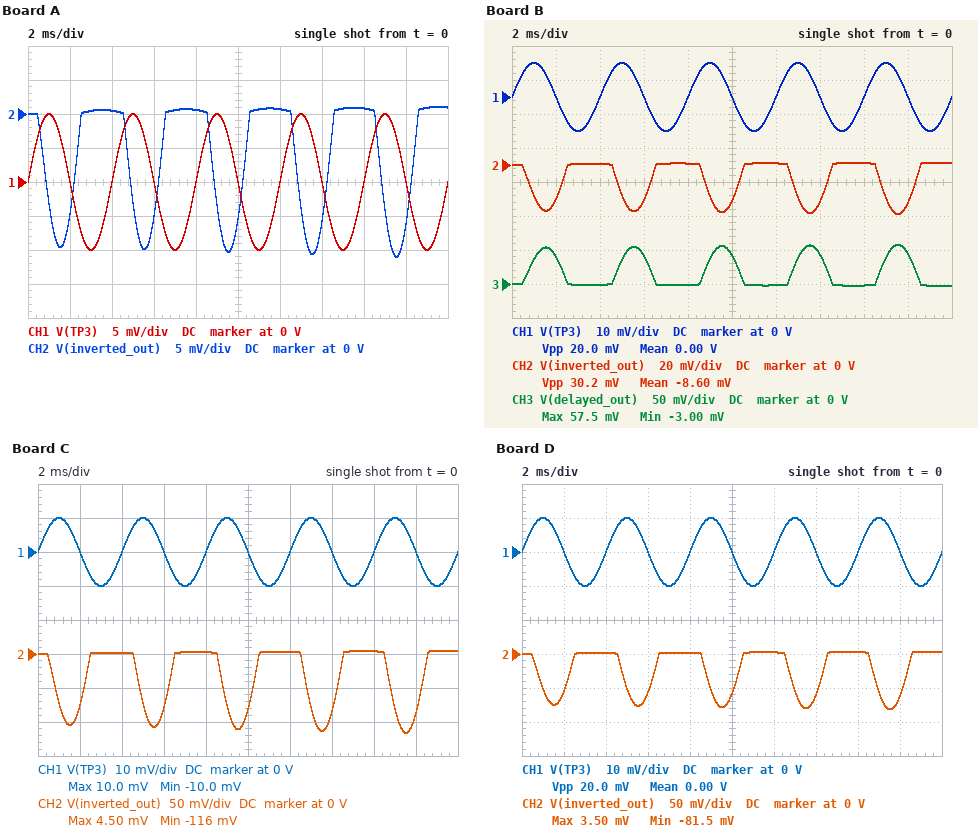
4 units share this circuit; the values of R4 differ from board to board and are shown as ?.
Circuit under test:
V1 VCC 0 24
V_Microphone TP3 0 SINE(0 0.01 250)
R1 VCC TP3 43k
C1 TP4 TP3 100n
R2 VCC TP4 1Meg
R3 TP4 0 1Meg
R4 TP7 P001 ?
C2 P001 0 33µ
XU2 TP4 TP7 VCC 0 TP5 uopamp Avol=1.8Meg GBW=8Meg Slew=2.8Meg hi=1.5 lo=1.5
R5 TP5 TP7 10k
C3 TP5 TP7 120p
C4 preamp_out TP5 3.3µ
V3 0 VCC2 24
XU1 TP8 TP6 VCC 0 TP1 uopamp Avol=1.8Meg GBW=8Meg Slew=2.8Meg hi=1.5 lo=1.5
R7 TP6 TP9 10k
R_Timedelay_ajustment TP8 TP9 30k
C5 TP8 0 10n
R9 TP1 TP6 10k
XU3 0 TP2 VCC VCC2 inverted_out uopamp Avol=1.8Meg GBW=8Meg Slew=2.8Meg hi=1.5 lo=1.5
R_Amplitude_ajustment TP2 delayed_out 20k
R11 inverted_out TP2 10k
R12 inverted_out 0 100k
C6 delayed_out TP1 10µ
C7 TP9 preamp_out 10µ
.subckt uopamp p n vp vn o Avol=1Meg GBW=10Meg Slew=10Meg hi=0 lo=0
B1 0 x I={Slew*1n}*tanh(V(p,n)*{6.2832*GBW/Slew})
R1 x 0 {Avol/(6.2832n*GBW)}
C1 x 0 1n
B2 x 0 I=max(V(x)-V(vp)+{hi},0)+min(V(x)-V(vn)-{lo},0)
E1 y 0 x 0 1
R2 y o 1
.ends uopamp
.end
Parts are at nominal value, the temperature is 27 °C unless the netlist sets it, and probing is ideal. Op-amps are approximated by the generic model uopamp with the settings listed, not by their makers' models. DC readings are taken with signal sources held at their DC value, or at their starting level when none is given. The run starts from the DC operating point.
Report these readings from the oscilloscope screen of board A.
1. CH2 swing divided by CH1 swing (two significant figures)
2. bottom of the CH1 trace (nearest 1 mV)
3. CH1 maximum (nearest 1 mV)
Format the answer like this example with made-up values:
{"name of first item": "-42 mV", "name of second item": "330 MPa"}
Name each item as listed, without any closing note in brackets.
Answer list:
{"CH2 swing divided by CH1 swing": "1.1", "bottom of the CH1 trace": "-10 mV", "CH1 maximum": "10 mV"}
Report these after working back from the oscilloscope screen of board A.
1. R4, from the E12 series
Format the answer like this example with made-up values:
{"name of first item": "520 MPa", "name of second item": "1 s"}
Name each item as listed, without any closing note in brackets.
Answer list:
{"R4, from the E12 series": "3.3 kΩ"}
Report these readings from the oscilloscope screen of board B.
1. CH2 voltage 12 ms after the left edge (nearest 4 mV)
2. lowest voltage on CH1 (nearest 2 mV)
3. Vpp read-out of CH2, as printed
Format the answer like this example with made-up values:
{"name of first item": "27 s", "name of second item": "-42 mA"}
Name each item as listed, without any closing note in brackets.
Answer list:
{"CH2 voltage 12 ms after the left edge": "0 V", "lowest voltage on CH1": "-10 mV", "Vpp read-out of CH2, as printed": "30.2 mV"}
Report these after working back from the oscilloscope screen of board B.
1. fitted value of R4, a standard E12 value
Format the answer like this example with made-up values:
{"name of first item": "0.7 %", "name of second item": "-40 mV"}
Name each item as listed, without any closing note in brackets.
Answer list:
{"fitted value of R4, a standard E12 value": "2.2 kΩ"}
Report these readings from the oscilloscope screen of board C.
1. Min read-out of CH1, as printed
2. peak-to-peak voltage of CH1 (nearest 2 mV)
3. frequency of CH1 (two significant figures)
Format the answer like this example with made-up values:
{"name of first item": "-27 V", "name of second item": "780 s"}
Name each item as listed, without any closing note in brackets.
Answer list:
{"Min read-out of CH1, as printed": "-10.0 mV", "peak-to-peak voltage of CH1": "20 mV", "frequency of CH1": "250 Hz"}
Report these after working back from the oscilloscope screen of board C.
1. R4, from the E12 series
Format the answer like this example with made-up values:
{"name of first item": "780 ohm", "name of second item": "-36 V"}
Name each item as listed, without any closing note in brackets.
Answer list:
{"R4, from the E12 series": "470 Ω"}
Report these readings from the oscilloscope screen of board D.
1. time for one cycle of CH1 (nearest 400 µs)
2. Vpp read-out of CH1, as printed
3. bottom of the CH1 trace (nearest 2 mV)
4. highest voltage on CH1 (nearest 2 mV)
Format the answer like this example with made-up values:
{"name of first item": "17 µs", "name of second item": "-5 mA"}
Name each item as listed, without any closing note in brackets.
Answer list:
{"time for one cycle of CH1": "4.0 ms", "Vpp read-out of CH1, as printed": "20.0 mV", "bottom of the CH1 trace": "-10 mV", "highest voltage on CH1": "10 mV"}
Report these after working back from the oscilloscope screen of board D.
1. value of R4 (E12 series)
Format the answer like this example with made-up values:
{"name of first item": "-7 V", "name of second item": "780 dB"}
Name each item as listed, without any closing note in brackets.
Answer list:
{"value of R4": "680 Ω"}
